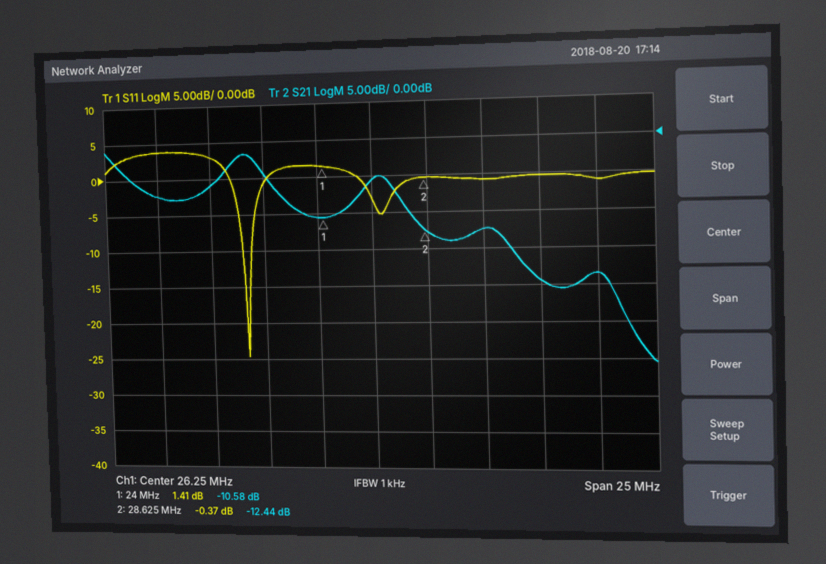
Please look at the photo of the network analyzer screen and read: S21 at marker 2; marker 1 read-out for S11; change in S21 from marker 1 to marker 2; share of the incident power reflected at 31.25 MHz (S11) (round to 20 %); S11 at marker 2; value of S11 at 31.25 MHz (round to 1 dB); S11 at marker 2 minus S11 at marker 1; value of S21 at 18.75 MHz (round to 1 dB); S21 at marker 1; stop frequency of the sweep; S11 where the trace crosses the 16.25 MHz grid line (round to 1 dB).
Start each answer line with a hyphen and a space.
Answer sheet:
- -12.44 dB
- 1.41 dB
- -1.86 dB
- 80 %
- -0.37 dB
- -1 dB
- -1.78 dB
- -6 dB
- -10.58 dB
- 38.75 MHz
- 4 dB
